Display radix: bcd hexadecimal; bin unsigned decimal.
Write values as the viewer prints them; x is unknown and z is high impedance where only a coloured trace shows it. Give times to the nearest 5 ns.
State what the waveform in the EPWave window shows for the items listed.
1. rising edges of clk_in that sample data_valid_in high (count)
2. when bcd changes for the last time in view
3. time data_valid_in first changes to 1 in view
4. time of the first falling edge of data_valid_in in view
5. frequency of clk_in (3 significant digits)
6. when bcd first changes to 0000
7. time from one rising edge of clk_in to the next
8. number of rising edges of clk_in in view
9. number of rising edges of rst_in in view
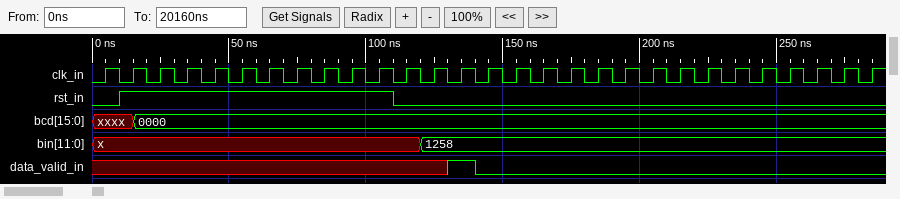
1
15 ns
130 ns
140 ns
100 MHz
15 ns
10 ns
29
1
